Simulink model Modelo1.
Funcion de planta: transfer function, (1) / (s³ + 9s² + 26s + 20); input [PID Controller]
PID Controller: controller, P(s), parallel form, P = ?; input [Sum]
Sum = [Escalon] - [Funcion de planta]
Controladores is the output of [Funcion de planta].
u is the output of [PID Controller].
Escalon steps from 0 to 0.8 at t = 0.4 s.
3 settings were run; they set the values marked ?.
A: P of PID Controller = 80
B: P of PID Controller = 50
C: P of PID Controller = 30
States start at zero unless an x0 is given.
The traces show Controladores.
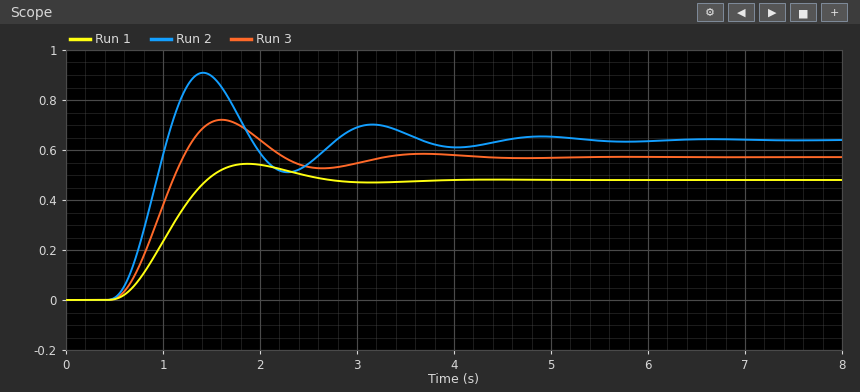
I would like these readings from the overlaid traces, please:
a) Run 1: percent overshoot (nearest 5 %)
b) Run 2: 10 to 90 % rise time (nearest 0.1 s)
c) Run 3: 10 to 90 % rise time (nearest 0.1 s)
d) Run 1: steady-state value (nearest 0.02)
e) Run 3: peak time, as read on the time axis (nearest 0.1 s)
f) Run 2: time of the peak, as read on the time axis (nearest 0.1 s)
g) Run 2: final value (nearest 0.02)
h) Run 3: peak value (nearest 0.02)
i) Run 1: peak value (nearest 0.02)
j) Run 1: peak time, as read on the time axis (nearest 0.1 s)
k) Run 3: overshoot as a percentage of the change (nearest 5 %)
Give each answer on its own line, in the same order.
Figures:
15 %
0.4 s
0.5 s
0.48
1.6 s
1.4 s
0.64
0.72
0.54
1.9 s
25 %
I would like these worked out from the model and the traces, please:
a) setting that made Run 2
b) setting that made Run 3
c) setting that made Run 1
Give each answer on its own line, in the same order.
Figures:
A
B
C
